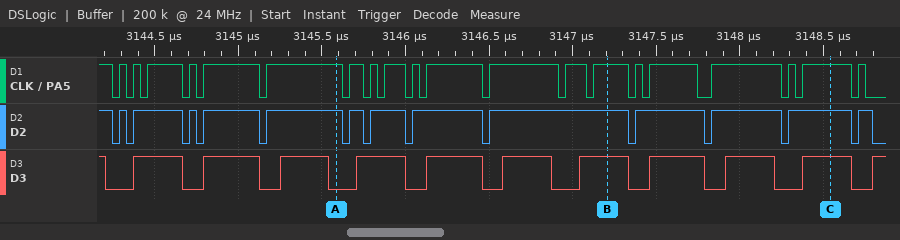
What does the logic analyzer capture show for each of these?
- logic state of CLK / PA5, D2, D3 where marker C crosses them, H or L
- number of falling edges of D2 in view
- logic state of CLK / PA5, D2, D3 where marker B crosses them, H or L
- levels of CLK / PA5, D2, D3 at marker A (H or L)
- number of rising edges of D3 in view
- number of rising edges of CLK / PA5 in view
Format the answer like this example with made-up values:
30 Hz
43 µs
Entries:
CLK / PA5=H, D2=H, D3=H
14
CLK / PA5=H, D2=H, D3=H
CLK / PA5=H, D2=H, D3=L
11
20
